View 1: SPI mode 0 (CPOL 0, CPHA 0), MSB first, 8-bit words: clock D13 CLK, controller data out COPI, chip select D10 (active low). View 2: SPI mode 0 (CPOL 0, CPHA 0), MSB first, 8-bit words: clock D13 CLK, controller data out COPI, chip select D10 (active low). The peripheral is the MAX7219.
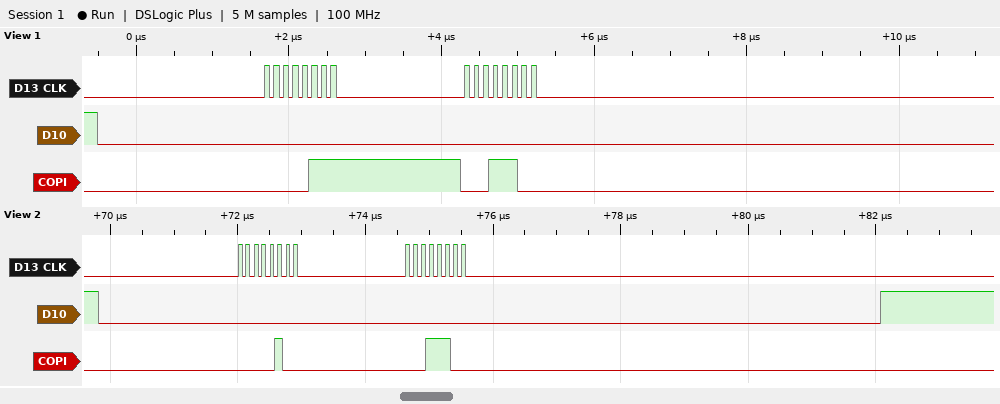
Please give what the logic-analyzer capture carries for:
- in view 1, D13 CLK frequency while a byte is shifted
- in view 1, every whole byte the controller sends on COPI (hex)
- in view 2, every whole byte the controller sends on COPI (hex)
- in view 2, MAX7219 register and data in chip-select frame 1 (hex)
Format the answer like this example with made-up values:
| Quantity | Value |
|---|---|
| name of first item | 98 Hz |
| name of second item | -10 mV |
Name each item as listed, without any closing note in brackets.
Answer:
| Quantity | Value |
|---|---|
| in view 1, D13 CLK frequency while a byte is shifted | 8 MHz |
| in view 1, every whole byte the controller sends on COPI | 07 1C |
| in view 2, every whole byte the controller sends on COPI | 04 1C |
| in view 2, MAX7219 register and data in chip-select frame 1 | register 0x4, data 0x1C |
